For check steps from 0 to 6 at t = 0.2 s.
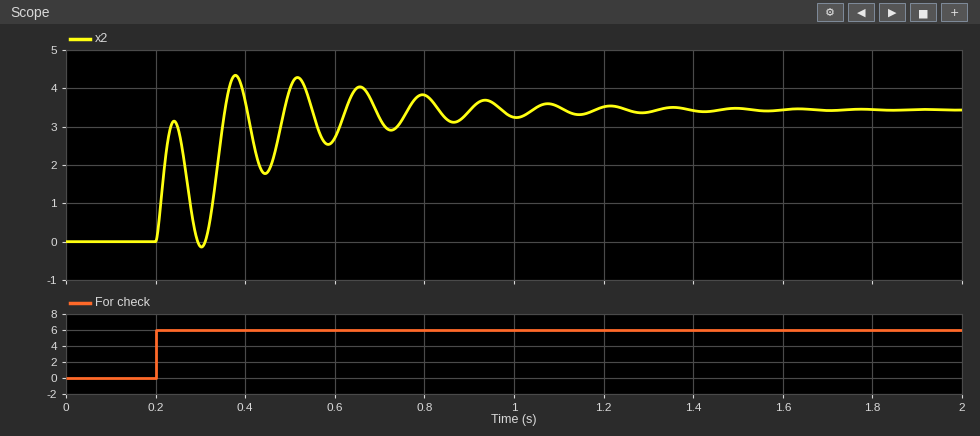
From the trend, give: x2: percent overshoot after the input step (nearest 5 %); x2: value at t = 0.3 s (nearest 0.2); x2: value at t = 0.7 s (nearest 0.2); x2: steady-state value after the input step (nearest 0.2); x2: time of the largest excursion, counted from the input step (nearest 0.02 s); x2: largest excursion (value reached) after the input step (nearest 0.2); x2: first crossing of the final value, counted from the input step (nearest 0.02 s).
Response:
25 %
-0.2
3.2
3.4
0.18 s
4.4
0.16 s
